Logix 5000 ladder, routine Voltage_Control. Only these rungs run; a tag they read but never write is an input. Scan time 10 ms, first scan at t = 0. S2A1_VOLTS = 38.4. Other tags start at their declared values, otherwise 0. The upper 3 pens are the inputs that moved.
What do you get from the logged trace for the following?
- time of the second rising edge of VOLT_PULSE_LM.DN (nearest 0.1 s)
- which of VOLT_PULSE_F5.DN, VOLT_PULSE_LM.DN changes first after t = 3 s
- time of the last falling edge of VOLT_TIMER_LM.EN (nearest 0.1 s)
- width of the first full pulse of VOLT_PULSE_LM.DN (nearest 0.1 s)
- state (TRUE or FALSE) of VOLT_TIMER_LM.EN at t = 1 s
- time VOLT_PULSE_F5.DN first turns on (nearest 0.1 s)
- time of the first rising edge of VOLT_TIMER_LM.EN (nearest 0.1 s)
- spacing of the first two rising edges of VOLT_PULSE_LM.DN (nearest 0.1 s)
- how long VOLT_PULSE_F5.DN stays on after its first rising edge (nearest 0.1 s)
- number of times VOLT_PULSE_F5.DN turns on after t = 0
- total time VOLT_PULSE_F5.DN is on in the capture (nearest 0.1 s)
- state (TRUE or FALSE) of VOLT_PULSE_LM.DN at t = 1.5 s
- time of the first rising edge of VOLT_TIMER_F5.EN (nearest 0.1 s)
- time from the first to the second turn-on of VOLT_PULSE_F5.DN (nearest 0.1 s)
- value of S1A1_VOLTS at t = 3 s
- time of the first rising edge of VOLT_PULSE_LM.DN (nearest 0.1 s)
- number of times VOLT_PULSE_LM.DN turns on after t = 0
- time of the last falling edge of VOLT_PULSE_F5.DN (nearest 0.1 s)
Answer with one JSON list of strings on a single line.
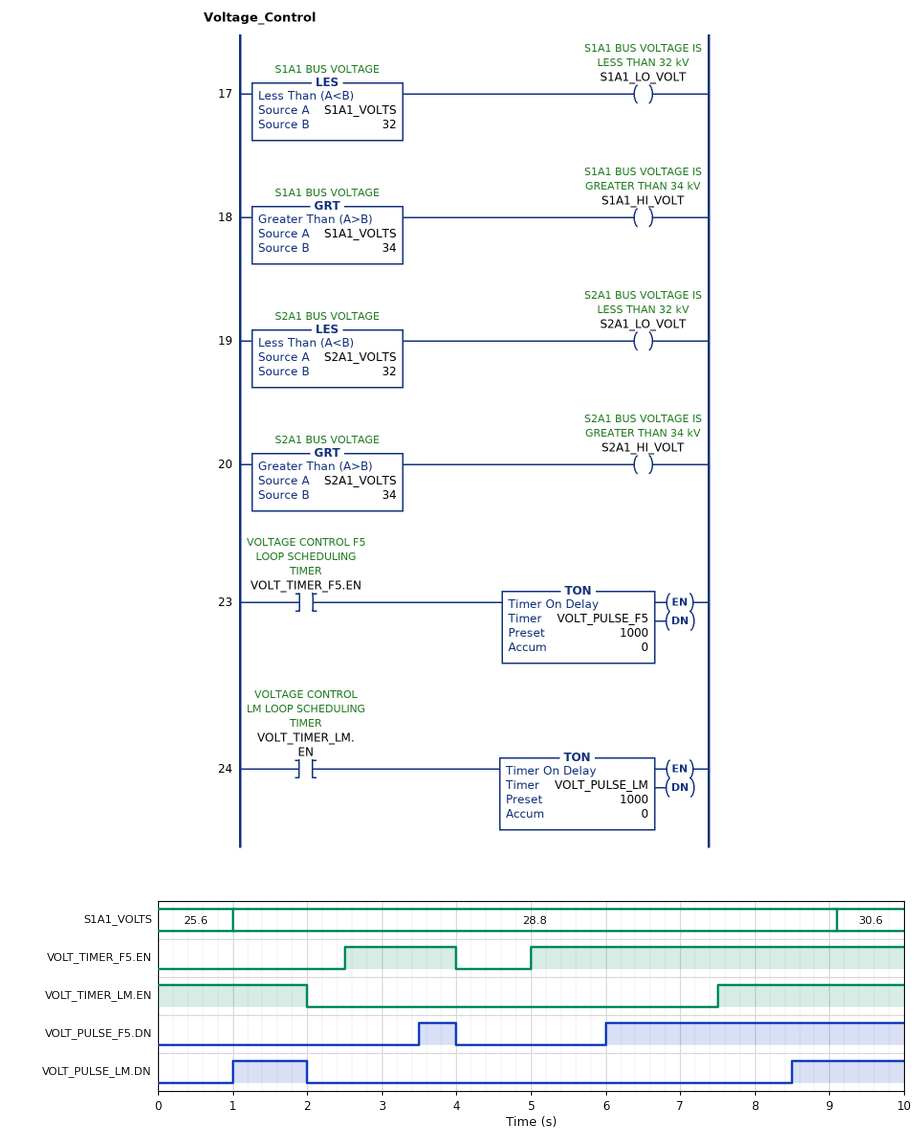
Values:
["8.5 s", "VOLT_PULSE_F5.DN", "2.0 s", "1.0 s", "TRUE", "3.5 s", "7.5 s", "7.5 s", "0.5 s", "2", "4.5 s", "TRUE", "2.5 s", "2.5 s", "28.8", "1.0 s", "2", "4.0 s"]
